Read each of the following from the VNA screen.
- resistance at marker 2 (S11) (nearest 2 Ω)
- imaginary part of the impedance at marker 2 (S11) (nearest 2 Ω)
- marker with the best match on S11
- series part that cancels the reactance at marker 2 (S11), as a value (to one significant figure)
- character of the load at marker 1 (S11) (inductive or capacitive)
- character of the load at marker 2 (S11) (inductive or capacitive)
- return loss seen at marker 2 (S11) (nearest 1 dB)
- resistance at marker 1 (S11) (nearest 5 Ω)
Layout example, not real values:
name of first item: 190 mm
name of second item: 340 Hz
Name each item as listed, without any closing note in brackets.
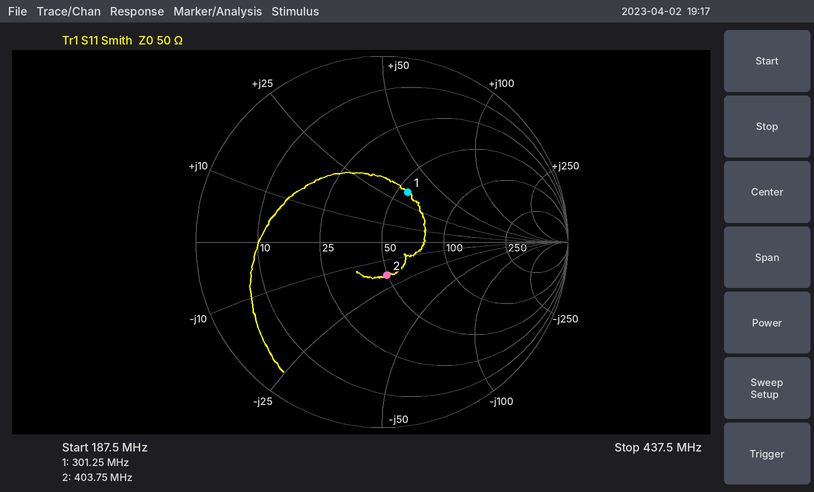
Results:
resistance at marker 2 (S11): 50 Ω
imaginary part of the impedance at marker 2 (S11): -18 Ω
marker with the best match on S11: marker 2
series part that cancels the reactance at marker 2 (S11), as a value: 7 nH
character of the load at marker 1 (S11): inductive
character of the load at marker 2 (S11): capacitive
return loss seen at marker 2 (S11): 15 dB
resistance at marker 1 (S11): 55 Ω
